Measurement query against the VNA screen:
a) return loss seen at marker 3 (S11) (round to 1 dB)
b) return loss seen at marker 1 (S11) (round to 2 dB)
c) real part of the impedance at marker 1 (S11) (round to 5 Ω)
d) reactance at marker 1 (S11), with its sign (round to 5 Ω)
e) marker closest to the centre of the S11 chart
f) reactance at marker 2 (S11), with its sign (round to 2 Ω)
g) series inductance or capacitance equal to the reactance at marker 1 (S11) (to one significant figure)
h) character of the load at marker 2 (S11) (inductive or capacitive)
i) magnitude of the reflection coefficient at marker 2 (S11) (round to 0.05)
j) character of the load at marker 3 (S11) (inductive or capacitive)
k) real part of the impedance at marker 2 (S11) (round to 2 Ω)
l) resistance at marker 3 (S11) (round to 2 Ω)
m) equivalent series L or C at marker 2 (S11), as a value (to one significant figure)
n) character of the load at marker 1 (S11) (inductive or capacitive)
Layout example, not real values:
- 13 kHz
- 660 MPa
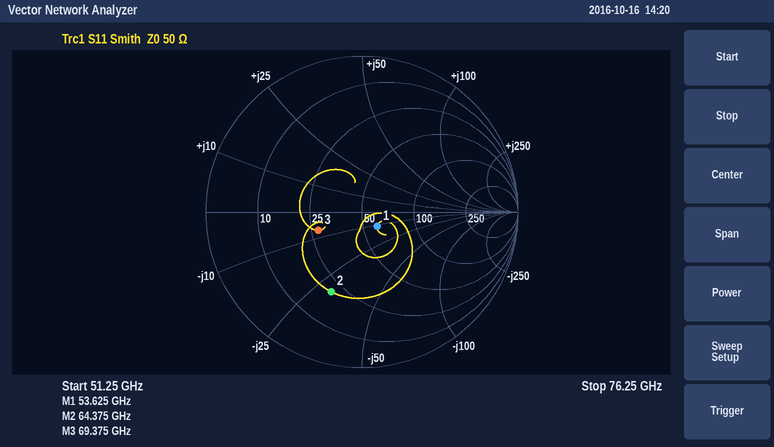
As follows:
- 10 dB
- 18 dB
- 60 Ω
- -10 Ω
- marker 1
- -30 Ω
- 300 fF
- capacitive
- 0.55
- capacitive
- 20 Ω
- 28 Ω
- 80 fF
- capacitive
